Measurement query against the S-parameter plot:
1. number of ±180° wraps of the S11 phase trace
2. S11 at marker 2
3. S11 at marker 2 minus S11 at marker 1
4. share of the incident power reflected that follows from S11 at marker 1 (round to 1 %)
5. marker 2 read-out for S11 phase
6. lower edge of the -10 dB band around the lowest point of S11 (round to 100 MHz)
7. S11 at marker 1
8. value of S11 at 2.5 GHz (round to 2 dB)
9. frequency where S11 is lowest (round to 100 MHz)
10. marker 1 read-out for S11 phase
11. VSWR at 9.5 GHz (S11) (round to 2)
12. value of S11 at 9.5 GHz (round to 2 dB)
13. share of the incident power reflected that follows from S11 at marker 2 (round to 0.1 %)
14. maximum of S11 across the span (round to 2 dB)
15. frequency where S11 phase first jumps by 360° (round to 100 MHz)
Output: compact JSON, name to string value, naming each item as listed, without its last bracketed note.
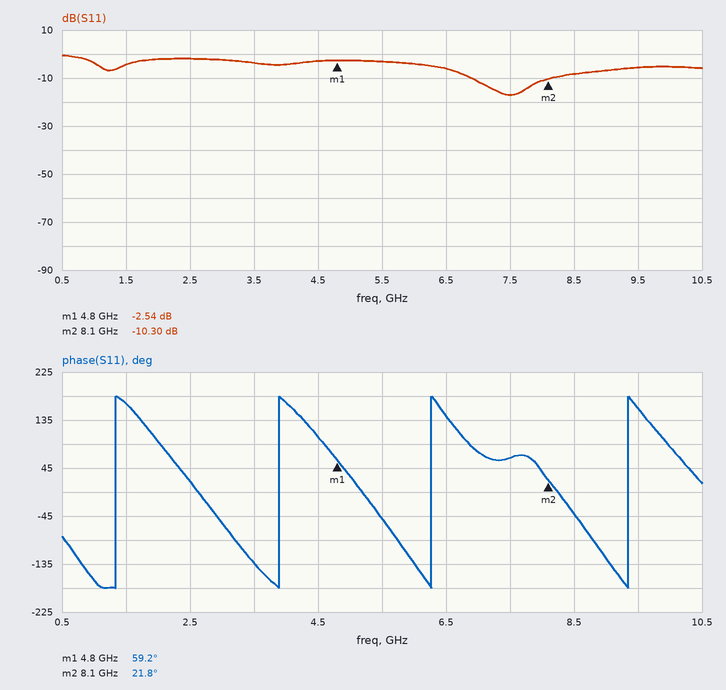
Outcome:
{"number of ±180° wraps of the S11 phase trace": "4", "S11 at marker 2": "-10.30 dB", "S11 at marker 2 minus S11 at marker 1": "-7.76 dB", "share of the incident power reflected that follows from S11 at marker 1": "56 %", "marker 2 read-out for S11 phase": "21.8°", "lower edge of the -10 dB band around the lowest point of S11": "6.9 GHz", "S11 at marker 1": "-2.54 dB", "value of S11 at 2.5 GHz": "-2 dB", "frequency where S11 is lowest": "7.5 GHz", "marker 1 read-out for S11 phase": "59.2°", "VSWR at 9.5 GHz (S11)": "4", "value of S11 at 9.5 GHz": "-6 dB", "share of the incident power reflected that follows from S11 at marker 2": "9.3 %", "maximum of S11 across the span": "0 dB", "frequency where S11 phase first jumps by 360°": "1.3 GHz"}
